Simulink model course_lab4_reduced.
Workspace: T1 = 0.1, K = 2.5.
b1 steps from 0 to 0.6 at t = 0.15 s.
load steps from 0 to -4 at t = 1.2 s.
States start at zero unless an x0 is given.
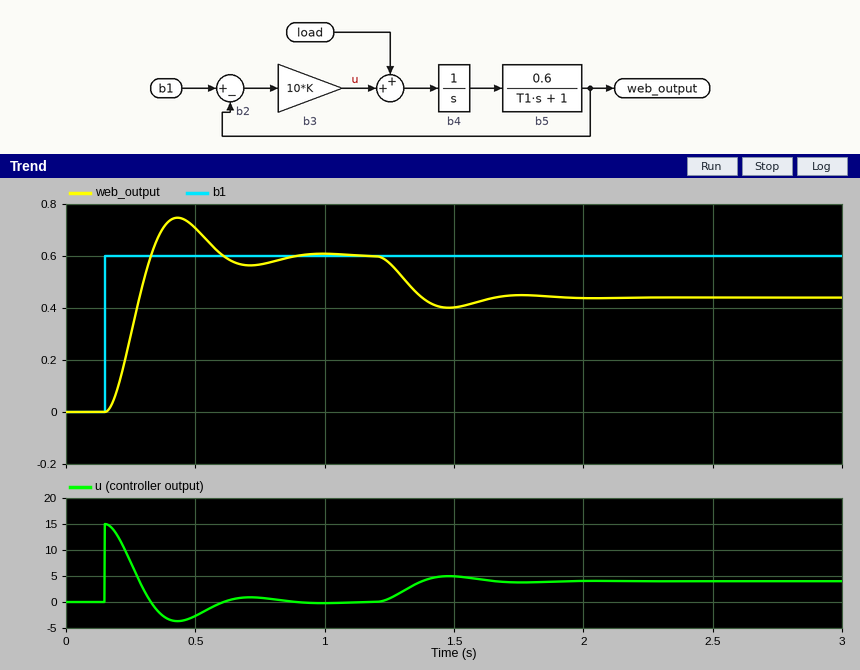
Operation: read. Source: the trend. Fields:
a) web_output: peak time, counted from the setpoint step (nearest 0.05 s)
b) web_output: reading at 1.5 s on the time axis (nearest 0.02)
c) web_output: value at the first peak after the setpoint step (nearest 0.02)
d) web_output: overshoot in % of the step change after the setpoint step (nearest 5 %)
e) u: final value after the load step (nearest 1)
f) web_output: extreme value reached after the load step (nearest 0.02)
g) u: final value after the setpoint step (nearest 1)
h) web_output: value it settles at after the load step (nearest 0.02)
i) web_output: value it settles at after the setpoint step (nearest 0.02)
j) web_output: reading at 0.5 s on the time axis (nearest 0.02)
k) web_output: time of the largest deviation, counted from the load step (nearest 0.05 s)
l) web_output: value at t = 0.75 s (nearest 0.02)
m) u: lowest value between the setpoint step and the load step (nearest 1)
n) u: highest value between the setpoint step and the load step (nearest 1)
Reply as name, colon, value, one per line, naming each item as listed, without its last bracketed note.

web_output: peak time, counted from the setpoint step: 0.30 s
web_output: reading at 1.5 s on the time axis: 0.40
web_output: value at the first peak after the setpoint step: 0.74
web_output: overshoot in % of the step change after the setpoint step: 25 %
u: final value after the load step: 4
web_output: extreme value reached after the load step: 0.40
u: final value after the setpoint step: 0
web_output: value it settles at after the load step: 0.44
web_output: value it settles at after the setpoint step: 0.60
web_output: reading at 0.5 s on the time axis: 0.70
web_output: time of the largest deviation, counted from the load step: 0.30 s
web_output: value at t = 0.75 s: 0.56
u: lowest value between the setpoint step and the load step: -4
u: highest value between the setpoint step and the load step: 15
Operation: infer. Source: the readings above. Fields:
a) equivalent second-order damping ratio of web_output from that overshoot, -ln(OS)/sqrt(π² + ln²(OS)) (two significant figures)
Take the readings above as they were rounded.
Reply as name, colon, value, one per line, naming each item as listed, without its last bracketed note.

equivalent second-order damping ratio of web_output from that overshoot, -ln(OS)/sqrt(π² + ln²(OS)): 0.40
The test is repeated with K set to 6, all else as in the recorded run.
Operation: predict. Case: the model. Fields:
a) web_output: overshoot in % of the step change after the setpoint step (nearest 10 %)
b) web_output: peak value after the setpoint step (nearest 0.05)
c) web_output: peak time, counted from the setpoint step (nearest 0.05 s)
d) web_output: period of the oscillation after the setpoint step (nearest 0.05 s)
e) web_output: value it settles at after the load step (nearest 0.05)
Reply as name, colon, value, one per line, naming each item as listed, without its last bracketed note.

web_output: overshoot in % of the step change after the setpoint step: 40 %
web_output: peak value after the setpoint step: 0.85
web_output: peak time, counted from the setpoint step: 0.15 s
web_output: period of the oscillation after the setpoint step: 0.35 s
web_output: value it settles at after the load step: 0.55
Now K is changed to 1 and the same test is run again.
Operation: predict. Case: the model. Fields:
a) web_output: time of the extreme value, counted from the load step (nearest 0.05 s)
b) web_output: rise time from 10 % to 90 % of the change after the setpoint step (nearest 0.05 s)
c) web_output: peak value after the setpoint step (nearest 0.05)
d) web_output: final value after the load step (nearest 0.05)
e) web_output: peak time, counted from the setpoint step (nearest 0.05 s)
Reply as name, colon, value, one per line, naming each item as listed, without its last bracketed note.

web_output: time of the extreme value, counted from the load step: 0.55 s
web_output: rise time from 10 % to 90 % of the change after the setpoint step: 0.25 s
web_output: peak value after the setpoint step: 0.65
web_output: final value after the load step: 0.20
web_output: peak time, counted from the setpoint step: 0.55 s
